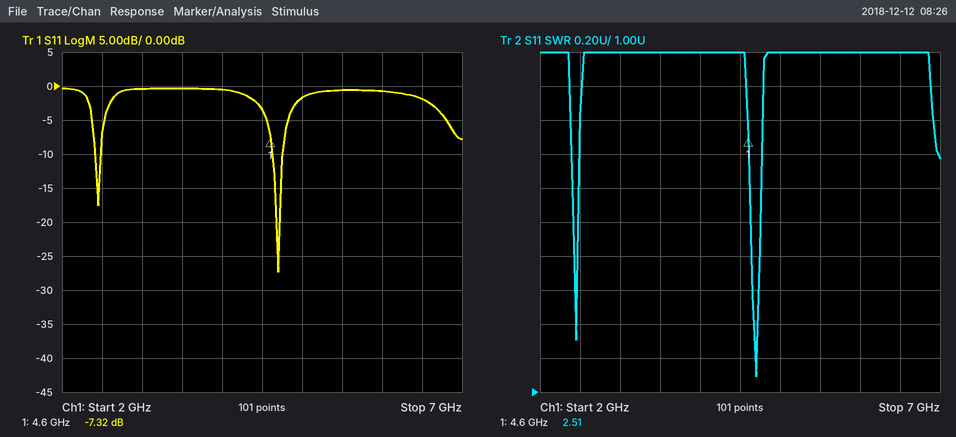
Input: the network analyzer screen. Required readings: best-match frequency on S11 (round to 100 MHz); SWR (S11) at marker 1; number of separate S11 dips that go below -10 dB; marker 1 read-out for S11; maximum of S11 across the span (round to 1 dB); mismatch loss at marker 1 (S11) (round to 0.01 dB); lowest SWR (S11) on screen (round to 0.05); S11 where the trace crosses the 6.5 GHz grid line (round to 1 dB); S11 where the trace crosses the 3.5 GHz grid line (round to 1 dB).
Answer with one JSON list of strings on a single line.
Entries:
["4.7 GHz", "2.51", "2", "-7.32 dB", "0 dB", "0.89 dB", "1.10", "-2 dB", "0 dB"]
